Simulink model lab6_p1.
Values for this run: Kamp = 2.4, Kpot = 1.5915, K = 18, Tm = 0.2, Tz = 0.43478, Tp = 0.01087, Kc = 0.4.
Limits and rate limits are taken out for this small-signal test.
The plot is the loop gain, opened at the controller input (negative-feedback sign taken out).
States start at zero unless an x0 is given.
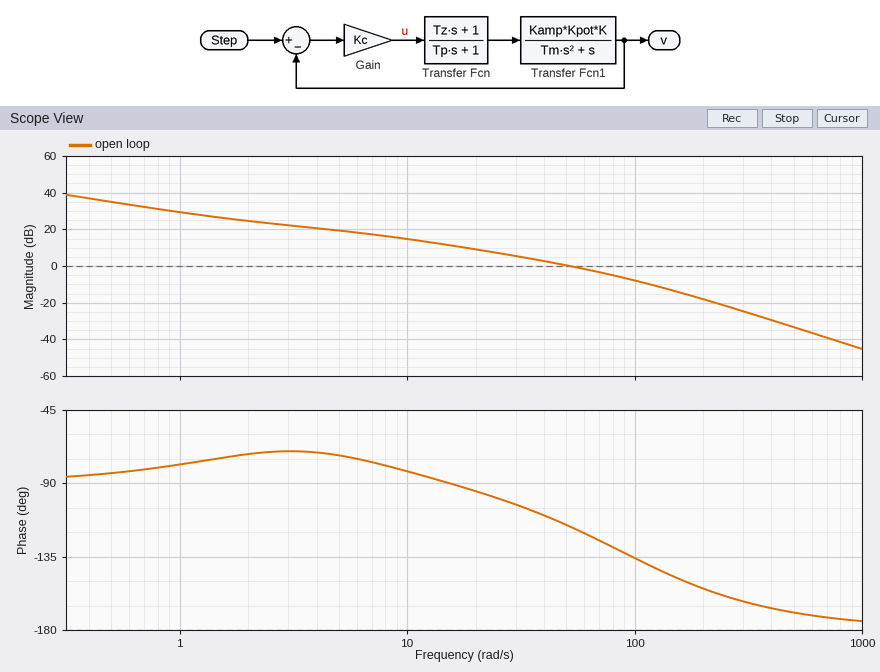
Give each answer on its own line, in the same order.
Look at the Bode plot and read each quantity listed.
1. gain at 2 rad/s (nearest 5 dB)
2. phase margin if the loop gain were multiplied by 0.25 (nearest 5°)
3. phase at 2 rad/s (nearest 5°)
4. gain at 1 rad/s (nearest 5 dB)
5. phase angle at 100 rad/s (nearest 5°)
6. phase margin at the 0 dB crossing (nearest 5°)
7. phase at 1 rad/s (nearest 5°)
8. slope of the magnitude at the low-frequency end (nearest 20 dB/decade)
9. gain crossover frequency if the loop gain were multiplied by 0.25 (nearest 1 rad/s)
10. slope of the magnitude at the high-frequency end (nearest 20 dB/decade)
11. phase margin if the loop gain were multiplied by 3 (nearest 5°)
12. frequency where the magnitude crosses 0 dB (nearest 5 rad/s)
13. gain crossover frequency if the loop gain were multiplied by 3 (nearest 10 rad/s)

25 dB
90°
-70°
30 dB
-135°
65°
-80°
-20 dB/decade
14 rad/s
-40 dB/decade
40°
50 rad/s
110 rad/s
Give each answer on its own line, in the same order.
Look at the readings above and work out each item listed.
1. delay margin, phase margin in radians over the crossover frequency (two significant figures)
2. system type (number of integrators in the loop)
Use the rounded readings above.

0.023 s
1
